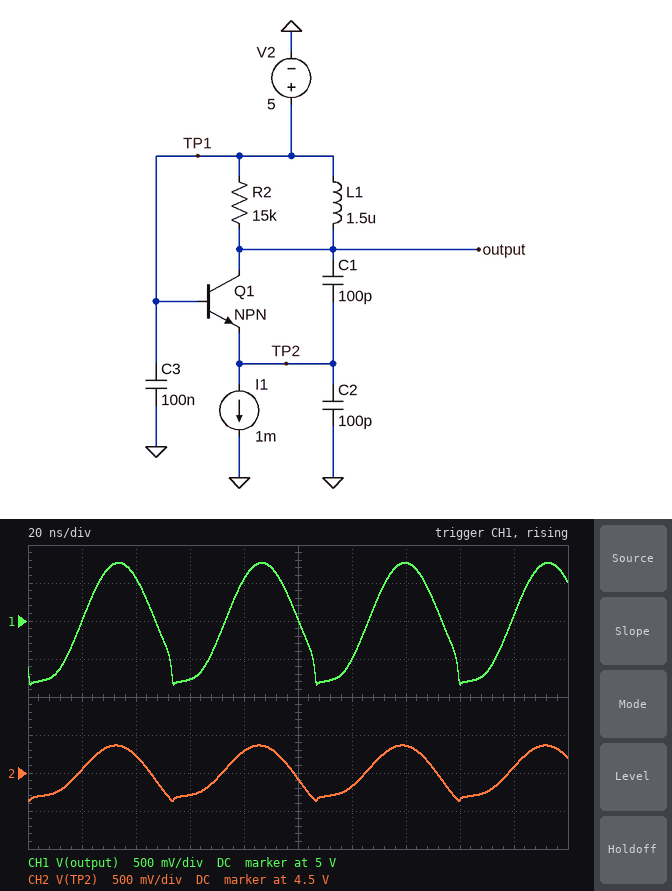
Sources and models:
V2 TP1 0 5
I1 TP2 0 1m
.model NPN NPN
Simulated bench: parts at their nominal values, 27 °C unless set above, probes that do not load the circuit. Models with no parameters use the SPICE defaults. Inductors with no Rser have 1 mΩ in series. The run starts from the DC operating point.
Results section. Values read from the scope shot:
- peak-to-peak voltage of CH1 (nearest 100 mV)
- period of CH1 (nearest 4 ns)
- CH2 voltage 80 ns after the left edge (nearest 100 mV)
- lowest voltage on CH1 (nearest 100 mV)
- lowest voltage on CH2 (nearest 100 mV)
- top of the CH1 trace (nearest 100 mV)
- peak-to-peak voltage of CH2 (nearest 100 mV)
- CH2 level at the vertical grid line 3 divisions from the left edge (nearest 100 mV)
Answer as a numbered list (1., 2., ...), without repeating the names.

1. 1.6 V
2. 52 ns
3. 4.8 V
4. 4.2 V
5. 4.1 V
6. 5.8 V
7. 700 mV
8. 4.2 V
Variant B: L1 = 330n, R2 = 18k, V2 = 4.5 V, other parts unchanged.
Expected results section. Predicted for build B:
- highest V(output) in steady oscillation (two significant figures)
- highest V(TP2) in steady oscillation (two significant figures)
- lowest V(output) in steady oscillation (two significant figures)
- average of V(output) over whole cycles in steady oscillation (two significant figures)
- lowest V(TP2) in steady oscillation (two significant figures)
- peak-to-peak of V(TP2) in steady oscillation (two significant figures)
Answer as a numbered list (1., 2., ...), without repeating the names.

1. 5.3 V
2. 4.4 V
3. 3.7 V
4. 4.5 V
5. 3.6 V
6. 790 mV
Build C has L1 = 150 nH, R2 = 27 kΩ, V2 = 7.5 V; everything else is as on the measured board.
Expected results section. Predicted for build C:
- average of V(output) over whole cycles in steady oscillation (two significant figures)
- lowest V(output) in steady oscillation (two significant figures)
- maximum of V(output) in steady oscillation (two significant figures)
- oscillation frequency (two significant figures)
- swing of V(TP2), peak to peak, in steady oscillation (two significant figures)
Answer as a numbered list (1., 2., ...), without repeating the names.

1. 7.5 V
2. 6.7 V
3. 8.3 V
4. 58 MHz
5. 800 mV
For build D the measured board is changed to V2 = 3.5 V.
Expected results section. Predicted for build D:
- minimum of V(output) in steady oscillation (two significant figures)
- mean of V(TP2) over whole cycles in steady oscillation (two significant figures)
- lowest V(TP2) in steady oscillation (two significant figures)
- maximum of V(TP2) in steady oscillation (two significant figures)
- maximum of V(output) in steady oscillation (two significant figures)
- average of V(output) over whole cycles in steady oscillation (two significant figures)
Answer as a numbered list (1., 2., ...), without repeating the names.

1. 2.7 V
2. 3.0 V
3. 2.6 V
4. 3.4 V
5. 4.3 V
6. 3.5 V
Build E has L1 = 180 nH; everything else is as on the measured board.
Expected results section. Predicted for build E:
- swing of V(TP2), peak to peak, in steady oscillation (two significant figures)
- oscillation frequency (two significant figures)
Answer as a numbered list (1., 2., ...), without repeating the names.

1. 800 mV
2. 53 MHz
